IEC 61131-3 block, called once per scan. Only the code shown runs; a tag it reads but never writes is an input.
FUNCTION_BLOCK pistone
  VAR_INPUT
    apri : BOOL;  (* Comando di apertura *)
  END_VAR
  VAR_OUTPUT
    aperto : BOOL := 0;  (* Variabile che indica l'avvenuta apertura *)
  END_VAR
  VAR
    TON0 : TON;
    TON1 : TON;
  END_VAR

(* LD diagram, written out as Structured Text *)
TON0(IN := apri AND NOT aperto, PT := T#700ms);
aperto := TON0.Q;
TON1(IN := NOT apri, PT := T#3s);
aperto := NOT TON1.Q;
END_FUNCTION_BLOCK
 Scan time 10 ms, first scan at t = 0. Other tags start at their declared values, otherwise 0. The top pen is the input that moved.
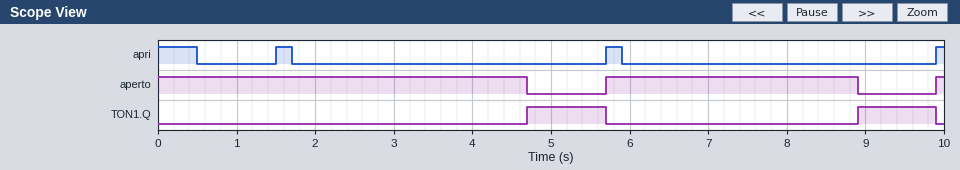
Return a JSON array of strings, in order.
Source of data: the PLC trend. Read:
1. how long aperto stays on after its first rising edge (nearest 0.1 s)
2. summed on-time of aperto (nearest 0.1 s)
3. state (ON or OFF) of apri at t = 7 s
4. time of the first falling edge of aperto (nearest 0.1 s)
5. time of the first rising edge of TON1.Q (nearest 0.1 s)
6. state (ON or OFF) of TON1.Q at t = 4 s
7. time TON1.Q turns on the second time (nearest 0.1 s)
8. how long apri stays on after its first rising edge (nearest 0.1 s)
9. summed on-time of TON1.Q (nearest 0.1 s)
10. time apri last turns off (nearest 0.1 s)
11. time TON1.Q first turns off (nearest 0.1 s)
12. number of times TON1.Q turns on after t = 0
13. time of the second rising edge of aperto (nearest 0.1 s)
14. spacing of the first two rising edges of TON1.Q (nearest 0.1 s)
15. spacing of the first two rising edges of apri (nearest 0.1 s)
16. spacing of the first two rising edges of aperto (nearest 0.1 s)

["3.2 s", "8.0 s", "OFF", "4.7 s", "4.7 s", "OFF", "8.9 s", "0.2 s", "2.0 s", "5.9 s", "5.7 s", "2", "9.9 s", "4.2 s", "4.2 s", "4.2 s"]
